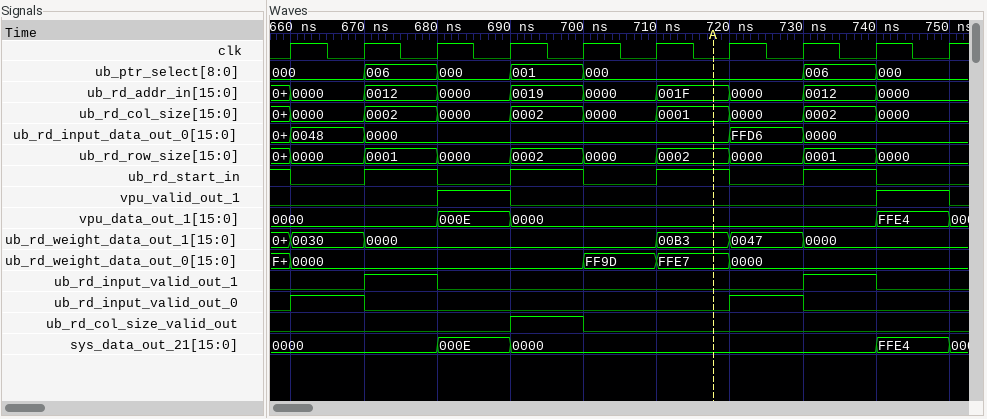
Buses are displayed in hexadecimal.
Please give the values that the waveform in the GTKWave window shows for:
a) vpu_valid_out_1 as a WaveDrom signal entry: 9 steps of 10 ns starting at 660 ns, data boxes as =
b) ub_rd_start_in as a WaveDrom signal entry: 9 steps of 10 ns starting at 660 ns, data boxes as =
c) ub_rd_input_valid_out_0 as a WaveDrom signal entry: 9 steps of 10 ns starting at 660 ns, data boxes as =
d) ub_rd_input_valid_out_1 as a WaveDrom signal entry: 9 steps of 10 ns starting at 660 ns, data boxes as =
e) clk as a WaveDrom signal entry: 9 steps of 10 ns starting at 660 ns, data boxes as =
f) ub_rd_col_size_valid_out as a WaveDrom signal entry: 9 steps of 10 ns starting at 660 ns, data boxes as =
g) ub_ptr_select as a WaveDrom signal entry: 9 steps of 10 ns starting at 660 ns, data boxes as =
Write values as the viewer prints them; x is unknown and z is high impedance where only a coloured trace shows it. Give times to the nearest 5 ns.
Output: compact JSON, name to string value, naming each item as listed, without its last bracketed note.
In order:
{"vpu_valid_out_1 as a WaveDrom signal entry: 9 steps of 10 ns starting at 660 ns, data boxes as =": "{name: 'vpu_valid_out_1', wave: '0.10....1'}", "ub_rd_start_in as a WaveDrom signal entry: 9 steps of 10 ns starting at 660 ns, data boxes as =": "{name: 'ub_rd_start_in', wave: '010101010'}", "ub_rd_input_valid_out_0 as a WaveDrom signal entry: 9 steps of 10 ns starting at 660 ns, data boxes as =": "{name: 'ub_rd_input_valid_out_0', wave: '10....10.'}", "ub_rd_input_valid_out_1 as a WaveDrom signal entry: 9 steps of 10 ns starting at 660 ns, data boxes as =": "{name: 'ub_rd_input_valid_out_1', wave: '010....10'}", "clk as a WaveDrom signal entry: 9 steps of 10 ns starting at 660 ns, data boxes as =": "{name: 'clk', wave: 'p........'}", "ub_rd_col_size_valid_out as a WaveDrom signal entry: 9 steps of 10 ns starting at 660 ns, data boxes as =": "{name: 'ub_rd_col_size_valid_out', wave: '0..10....'}", "ub_ptr_select as a WaveDrom signal entry: 9 steps of 10 ns starting at 660 ns, data boxes as =": "{name: 'ub_ptr_select', wave: '=====..==', data: '000 006 000 001 000 006 000'}"}
